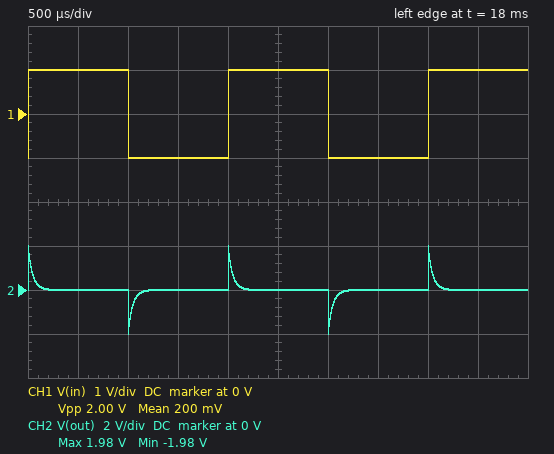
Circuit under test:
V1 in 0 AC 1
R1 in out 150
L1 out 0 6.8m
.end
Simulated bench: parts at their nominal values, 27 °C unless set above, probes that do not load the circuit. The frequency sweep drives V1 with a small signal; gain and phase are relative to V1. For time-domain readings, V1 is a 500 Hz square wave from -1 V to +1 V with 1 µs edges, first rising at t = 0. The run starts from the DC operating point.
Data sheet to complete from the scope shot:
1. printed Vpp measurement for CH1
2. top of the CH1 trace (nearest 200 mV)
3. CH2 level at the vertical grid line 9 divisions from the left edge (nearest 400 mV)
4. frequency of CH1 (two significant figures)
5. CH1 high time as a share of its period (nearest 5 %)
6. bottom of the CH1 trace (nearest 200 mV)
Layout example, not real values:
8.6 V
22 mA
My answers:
2.00 V
1.0 V
0 V
500 Hz
50 %
-1.0 V
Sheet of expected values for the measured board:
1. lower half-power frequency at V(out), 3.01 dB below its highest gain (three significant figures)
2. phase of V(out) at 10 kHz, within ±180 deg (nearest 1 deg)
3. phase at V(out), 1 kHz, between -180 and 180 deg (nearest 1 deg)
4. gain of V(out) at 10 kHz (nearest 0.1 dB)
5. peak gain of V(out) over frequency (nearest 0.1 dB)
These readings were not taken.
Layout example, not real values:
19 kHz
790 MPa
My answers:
3.51 kHz
19 deg
74 deg
-0.5 dB
0 dB
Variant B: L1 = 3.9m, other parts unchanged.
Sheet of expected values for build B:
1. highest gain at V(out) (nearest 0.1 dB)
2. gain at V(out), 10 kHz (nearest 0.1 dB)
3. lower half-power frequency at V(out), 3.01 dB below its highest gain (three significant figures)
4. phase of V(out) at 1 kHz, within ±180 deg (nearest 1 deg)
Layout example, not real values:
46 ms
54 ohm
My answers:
0 dB
-1.4 dB
6.12 kHz
81 deg
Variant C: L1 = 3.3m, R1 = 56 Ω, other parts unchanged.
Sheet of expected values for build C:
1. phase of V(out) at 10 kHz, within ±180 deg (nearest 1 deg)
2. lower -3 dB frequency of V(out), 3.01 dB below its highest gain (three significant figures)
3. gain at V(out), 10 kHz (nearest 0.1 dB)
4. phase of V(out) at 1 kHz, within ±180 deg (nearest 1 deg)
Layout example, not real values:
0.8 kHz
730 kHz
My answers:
15 deg
2.70 kHz
-0.3 dB
70 deg
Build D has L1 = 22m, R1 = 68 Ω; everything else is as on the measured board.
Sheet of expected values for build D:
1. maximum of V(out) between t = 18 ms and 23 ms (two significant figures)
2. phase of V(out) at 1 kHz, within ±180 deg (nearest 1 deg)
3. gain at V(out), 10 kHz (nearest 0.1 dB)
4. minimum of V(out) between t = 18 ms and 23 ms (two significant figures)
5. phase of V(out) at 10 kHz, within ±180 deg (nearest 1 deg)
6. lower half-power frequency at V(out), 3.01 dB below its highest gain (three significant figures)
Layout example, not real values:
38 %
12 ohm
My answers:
1.9 V
26 deg
0 dB
-1.9 V
3 deg
492 Hz
